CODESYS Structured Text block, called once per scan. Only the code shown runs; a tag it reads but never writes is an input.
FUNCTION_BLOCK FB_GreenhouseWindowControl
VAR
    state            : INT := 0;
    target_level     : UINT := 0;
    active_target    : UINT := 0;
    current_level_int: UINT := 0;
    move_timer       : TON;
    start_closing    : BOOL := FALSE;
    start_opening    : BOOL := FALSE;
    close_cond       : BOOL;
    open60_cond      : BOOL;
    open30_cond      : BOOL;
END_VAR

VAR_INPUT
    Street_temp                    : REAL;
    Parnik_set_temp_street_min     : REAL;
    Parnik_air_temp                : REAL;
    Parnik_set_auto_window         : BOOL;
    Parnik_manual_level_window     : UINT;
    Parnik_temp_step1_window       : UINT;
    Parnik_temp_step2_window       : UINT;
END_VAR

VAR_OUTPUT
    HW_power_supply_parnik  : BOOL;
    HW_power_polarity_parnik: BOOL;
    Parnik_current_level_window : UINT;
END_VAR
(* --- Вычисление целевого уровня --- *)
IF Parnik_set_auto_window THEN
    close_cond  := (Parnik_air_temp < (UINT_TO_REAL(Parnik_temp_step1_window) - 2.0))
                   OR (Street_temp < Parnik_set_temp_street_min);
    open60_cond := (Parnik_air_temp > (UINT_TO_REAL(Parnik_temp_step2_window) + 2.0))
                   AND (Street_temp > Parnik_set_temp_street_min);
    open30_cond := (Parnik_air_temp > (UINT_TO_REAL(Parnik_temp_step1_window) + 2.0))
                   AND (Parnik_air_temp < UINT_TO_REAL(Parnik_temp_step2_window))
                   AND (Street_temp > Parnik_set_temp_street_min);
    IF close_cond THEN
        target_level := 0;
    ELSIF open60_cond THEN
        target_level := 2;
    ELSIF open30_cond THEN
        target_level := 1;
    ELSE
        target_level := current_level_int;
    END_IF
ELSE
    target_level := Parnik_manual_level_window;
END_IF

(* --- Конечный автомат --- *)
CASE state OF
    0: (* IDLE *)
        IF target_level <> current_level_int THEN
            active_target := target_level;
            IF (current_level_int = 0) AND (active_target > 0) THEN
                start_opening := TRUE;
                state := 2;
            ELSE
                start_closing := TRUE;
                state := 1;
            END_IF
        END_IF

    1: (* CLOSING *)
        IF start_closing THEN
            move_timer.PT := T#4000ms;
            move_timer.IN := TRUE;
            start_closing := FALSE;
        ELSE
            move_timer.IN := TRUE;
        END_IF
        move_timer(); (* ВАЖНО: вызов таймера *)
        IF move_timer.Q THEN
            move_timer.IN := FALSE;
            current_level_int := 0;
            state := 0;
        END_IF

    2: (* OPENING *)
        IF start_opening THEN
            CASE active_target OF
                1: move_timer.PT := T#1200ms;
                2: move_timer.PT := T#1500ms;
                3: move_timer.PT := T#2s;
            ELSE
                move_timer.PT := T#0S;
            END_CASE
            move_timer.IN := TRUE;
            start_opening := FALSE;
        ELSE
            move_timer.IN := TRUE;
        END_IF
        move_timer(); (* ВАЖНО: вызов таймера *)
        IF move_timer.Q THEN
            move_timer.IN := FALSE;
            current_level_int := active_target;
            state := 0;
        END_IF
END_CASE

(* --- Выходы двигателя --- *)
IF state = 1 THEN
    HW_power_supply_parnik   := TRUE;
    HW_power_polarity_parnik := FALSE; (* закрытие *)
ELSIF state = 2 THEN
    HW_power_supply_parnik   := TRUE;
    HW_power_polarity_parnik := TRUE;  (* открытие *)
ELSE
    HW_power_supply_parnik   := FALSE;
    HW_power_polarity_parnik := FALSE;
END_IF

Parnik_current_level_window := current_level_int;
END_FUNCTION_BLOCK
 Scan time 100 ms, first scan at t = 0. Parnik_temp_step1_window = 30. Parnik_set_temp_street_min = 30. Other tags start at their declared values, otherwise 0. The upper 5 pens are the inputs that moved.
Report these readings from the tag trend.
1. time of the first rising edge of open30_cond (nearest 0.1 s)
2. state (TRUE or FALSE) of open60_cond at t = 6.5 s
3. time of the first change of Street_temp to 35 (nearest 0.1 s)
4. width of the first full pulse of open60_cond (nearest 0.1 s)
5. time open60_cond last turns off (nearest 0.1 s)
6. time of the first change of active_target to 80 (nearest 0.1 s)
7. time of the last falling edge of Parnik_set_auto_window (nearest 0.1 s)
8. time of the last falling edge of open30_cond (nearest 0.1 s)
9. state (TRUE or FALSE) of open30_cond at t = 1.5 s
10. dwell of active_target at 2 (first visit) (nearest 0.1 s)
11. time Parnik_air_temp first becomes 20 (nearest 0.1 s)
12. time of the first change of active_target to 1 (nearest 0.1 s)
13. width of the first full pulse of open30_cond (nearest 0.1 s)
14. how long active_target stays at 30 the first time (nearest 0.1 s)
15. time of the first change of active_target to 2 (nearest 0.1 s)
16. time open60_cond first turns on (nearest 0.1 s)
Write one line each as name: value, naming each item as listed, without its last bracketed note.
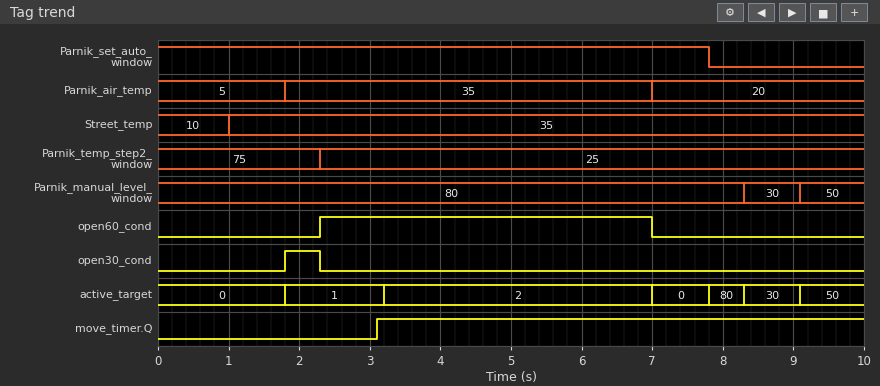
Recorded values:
time of the first rising edge of open30_cond: 1.8 s
state (TRUE or FALSE) of open60_cond at t = 6.5 s: TRUE
time of the first change of Street_temp to 35: 1.0 s
width of the first full pulse of open60_cond: 4.7 s
time open60_cond last turns off: 7.0 s
time of the first change of active_target to 80: 7.8 s
time of the last falling edge of Parnik_set_auto_window: 7.8 s
time of the last falling edge of open30_cond: 2.3 s
state (TRUE or FALSE) of open30_cond at t = 1.5 s: FALSE
dwell of active_target at 2 (first visit): 3.8 s
time Parnik_air_temp first becomes 20: 7.0 s
time of the first change of active_target to 1: 1.8 s
width of the first full pulse of open30_cond: 0.5 s
how long active_target stays at 30 the first time: 0.8 s
time of the first change of active_target to 2: 3.2 s
time open60_cond first turns on: 2.3 s
